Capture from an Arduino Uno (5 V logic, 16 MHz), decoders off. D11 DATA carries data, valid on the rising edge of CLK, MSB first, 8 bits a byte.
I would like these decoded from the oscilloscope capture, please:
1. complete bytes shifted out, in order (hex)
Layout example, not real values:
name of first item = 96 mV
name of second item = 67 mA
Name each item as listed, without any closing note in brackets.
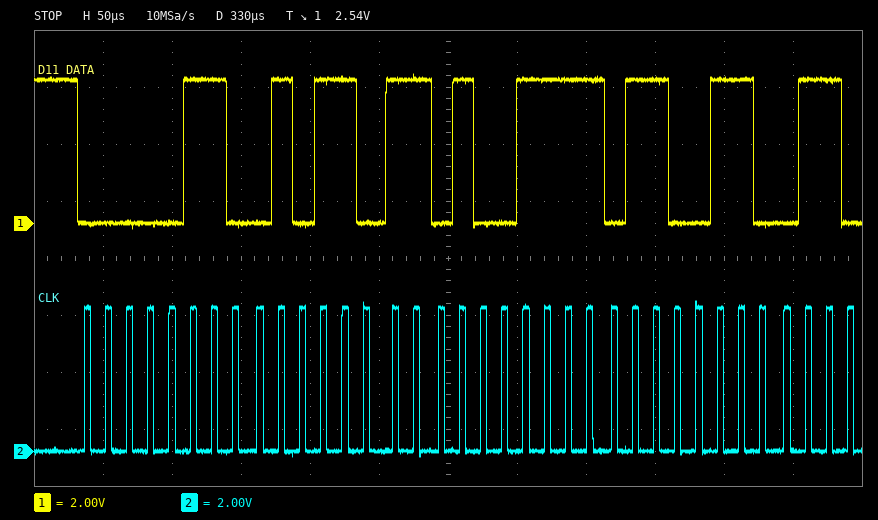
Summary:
complete bytes shifted out, in order = 0x06 0x5B 0x4F 0x66
